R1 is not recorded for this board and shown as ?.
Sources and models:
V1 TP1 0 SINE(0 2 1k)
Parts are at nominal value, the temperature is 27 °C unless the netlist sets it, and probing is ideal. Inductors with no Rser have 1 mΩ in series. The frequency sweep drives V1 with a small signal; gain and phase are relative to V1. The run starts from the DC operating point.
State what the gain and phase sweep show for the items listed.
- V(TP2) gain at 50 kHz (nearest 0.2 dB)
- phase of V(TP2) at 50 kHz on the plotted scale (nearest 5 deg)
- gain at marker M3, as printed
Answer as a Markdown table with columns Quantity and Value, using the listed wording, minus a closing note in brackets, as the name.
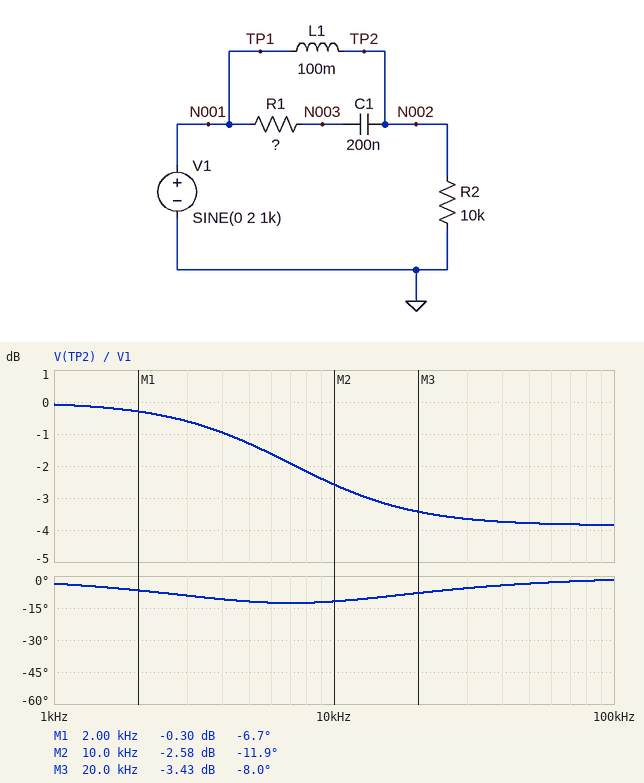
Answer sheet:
| Quantity | Value |
|---|---|
| V(TP2) gain at 50 kHz | -3.8 dB |
| phase of V(TP2) at 50 kHz on the plotted scale | -5 deg |
| gain at marker M3, as printed | -3.43 dB |
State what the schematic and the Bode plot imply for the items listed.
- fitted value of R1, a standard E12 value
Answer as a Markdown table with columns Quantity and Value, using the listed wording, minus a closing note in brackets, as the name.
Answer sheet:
| Quantity | Value |
|---|---|
| fitted value of R1, a standard E12 value | 5.6 kΩ |
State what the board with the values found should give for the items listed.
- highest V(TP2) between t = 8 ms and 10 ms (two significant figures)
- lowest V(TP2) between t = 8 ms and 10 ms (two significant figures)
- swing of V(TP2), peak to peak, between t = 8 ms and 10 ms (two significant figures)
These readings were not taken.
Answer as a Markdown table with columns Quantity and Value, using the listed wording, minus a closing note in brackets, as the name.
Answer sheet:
| Quantity | Value |
|---|---|
| highest V(TP2) between t = 8 ms and 10 ms | 2.0 V |
| lowest V(TP2) between t = 8 ms and 10 ms | -2.0 V |
| swing of V(TP2), peak to peak, between t = 8 ms and 10 ms | 4.0 V |
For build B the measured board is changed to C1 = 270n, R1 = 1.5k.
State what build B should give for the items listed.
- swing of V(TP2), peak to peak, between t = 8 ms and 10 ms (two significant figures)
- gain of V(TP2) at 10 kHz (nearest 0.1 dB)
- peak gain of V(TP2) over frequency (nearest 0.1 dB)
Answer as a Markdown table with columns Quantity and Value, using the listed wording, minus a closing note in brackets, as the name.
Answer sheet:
| Quantity | Value |
|---|---|
| swing of V(TP2), peak to peak, between t = 8 ms and 10 ms | 3.9 V |
| gain of V(TP2) at 10 kHz | -1.2 dB |
| peak gain of V(TP2) over frequency | 0 dB |
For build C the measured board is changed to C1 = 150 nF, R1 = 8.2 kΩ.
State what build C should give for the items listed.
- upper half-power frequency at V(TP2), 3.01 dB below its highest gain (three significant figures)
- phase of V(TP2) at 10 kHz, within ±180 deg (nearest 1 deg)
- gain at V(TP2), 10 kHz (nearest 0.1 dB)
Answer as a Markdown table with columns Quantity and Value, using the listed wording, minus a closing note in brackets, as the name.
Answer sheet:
| Quantity | Value |
|---|---|
| upper half-power frequency at V(TP2), 3.01 dB below its highest gain | 11.3 kHz |
| phase of V(TP2) at 10 kHz, within ±180 deg | -17 deg |
| gain at V(TP2), 10 kHz | -2.7 dB |
